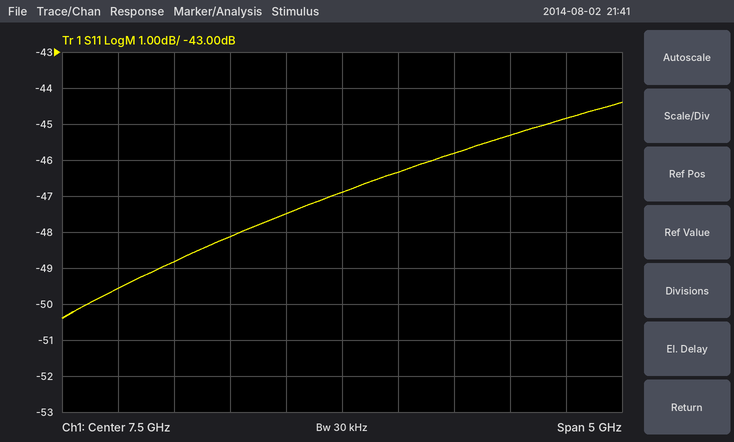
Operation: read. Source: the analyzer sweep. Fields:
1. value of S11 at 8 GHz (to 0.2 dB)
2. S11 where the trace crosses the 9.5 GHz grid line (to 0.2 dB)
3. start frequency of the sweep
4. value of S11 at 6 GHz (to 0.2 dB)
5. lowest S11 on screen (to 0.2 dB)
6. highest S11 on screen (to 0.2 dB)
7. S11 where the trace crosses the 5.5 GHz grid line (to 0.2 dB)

-46.4 dB
-44.8 dB
5 GHz
-48.8 dB
-50.4 dB
-44.4 dB
-49.6 dB
